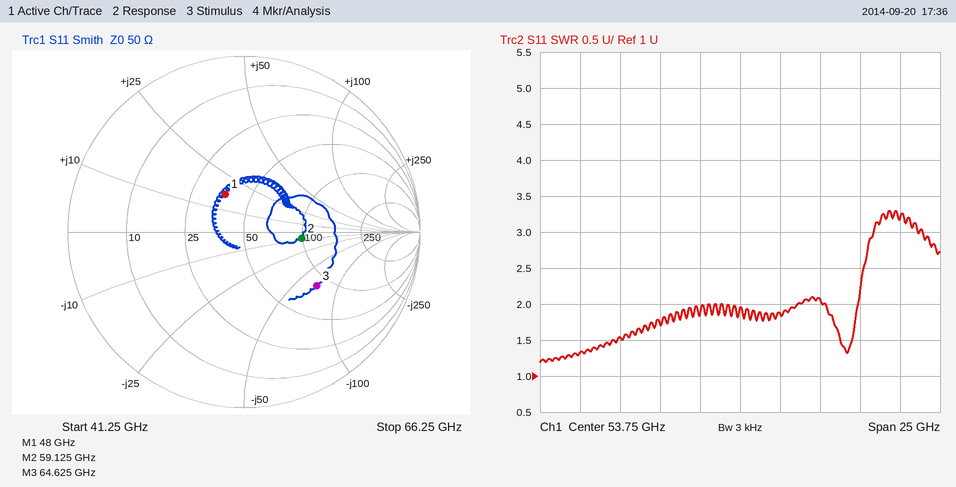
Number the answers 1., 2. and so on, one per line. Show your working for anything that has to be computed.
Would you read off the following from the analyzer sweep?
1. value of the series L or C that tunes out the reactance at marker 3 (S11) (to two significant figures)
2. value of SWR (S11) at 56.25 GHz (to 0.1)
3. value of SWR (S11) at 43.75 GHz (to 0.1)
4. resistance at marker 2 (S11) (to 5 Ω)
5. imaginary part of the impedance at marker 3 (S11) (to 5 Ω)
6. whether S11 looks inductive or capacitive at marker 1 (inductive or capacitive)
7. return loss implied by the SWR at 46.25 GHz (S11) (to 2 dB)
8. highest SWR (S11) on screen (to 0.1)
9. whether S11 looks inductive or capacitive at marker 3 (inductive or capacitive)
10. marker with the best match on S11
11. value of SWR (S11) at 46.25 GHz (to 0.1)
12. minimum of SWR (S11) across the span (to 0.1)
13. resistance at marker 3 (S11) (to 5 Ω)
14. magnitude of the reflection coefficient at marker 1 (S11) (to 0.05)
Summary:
1. L = 70 Ω/(2π × 64.625 GHz) ≈ 172 pH, so 170 pH to two significant figures
2. 1.9
3. 1.3
4. 100 Ω
5. -70 Ω
6. inductive
7. −20 log10((1.5 − 1)/(1.5 + 1)) ≈ 14 dB
8. 3.3
9. capacitive
10. marker 1
11. 1.5
12. 1.2
13. 85 Ω
14. 0.25
